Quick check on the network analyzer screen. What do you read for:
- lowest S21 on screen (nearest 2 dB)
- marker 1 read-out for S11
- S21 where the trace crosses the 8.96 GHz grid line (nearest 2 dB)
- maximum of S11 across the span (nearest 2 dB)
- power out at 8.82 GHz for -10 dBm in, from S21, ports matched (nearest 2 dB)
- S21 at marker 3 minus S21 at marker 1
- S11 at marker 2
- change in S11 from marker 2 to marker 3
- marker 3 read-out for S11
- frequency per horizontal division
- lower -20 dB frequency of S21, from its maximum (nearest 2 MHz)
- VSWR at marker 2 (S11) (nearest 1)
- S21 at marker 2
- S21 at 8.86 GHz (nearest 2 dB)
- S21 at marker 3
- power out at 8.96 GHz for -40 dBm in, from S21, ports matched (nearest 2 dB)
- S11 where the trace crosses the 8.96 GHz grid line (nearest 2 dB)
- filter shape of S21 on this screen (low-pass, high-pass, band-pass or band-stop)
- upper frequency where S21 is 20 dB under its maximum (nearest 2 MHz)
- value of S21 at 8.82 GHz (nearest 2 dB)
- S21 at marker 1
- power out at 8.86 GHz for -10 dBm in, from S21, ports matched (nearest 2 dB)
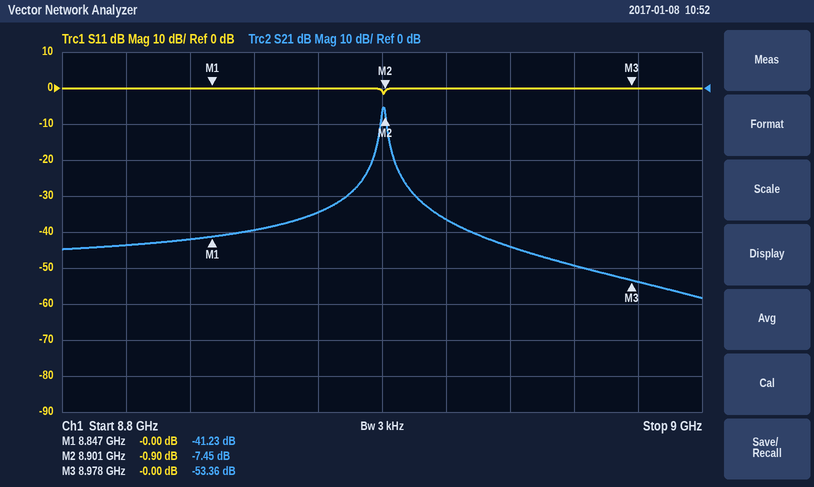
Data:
-58 dB
-0.00 dB
-50 dB
0 dB
-54 dBm
-12.13 dB
-0.90 dB
0.90 dB
-0.00 dB
20 MHz
8.894 GHz
19
-7.45 dB
-40 dB
-53.36 dB
-90 dBm
0 dB
band-pass
8.906 GHz
-44 dB
-41.23 dB
-50 dBm
